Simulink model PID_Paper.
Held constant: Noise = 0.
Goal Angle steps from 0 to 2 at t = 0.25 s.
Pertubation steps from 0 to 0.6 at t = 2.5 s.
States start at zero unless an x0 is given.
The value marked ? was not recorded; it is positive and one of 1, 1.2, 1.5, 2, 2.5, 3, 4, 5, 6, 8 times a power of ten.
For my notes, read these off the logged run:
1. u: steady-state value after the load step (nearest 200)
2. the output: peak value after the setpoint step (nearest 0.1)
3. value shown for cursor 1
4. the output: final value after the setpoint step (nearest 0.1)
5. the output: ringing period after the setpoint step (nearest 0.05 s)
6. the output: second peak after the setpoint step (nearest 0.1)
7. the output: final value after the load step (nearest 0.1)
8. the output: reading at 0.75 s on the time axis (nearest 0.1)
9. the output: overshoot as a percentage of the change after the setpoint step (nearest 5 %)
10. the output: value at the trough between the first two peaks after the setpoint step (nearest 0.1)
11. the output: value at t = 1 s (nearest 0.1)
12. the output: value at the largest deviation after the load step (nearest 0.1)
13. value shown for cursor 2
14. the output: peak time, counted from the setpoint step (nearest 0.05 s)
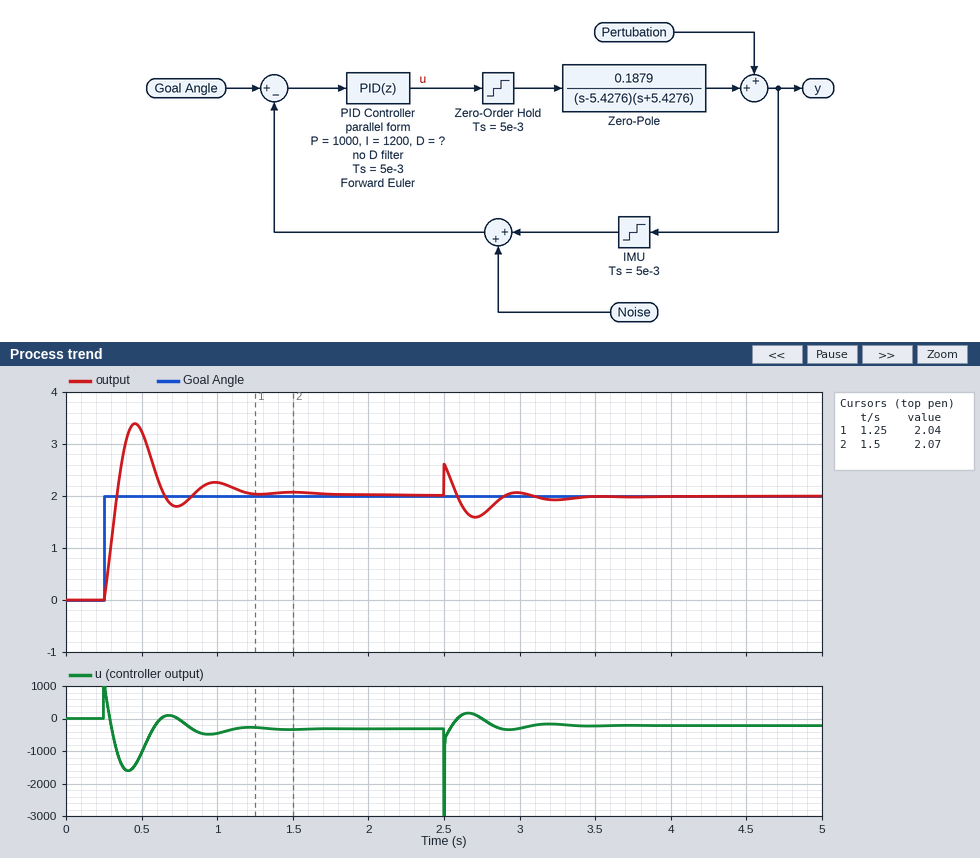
-200
3.4
2.04
2.0
0.55 s
2.3
2.0
1.8
70 %
1.8
2.3
2.6
2.07
0.20 s
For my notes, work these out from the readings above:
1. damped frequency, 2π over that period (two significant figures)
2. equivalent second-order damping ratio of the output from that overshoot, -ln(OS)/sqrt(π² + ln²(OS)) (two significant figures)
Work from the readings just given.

11 rad/s
0.11
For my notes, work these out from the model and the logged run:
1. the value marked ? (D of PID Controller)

50
